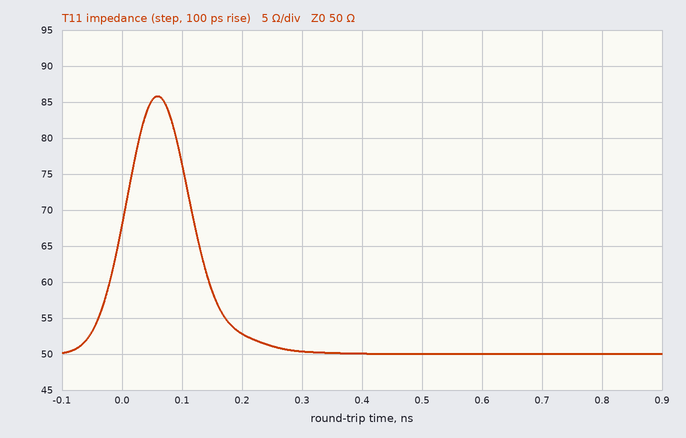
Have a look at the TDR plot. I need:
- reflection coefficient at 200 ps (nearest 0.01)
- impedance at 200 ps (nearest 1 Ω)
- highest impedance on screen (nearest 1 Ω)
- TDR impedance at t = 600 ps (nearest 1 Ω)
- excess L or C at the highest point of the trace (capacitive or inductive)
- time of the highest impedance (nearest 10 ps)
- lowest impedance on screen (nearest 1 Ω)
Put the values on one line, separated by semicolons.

+0.03; 53 Ω; 86 Ω; 50 Ω; inductive; 60 ps; 50 Ω
